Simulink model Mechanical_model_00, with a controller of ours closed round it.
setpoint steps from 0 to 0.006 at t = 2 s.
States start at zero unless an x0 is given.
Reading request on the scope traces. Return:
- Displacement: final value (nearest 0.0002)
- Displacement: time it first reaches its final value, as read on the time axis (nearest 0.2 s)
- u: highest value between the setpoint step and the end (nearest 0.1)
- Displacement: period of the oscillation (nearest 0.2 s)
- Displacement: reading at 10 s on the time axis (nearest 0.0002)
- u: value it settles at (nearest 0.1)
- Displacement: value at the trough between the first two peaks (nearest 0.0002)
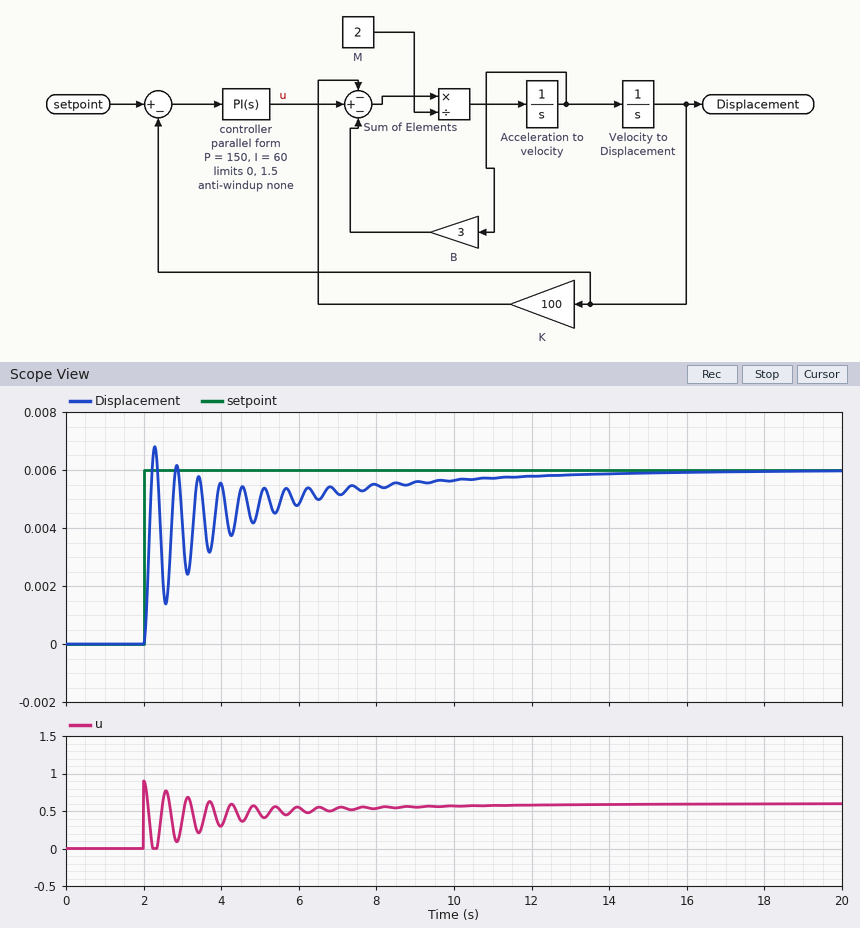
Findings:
0.0060
2.2 s
0.9
0.6 s
0.0056
0.6
0.0014
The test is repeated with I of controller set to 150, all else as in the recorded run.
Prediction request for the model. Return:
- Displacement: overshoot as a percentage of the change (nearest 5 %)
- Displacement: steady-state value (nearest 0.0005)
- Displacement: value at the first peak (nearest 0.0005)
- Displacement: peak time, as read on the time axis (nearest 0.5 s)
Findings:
20 %
0.0060
0.0070
2.5 s
